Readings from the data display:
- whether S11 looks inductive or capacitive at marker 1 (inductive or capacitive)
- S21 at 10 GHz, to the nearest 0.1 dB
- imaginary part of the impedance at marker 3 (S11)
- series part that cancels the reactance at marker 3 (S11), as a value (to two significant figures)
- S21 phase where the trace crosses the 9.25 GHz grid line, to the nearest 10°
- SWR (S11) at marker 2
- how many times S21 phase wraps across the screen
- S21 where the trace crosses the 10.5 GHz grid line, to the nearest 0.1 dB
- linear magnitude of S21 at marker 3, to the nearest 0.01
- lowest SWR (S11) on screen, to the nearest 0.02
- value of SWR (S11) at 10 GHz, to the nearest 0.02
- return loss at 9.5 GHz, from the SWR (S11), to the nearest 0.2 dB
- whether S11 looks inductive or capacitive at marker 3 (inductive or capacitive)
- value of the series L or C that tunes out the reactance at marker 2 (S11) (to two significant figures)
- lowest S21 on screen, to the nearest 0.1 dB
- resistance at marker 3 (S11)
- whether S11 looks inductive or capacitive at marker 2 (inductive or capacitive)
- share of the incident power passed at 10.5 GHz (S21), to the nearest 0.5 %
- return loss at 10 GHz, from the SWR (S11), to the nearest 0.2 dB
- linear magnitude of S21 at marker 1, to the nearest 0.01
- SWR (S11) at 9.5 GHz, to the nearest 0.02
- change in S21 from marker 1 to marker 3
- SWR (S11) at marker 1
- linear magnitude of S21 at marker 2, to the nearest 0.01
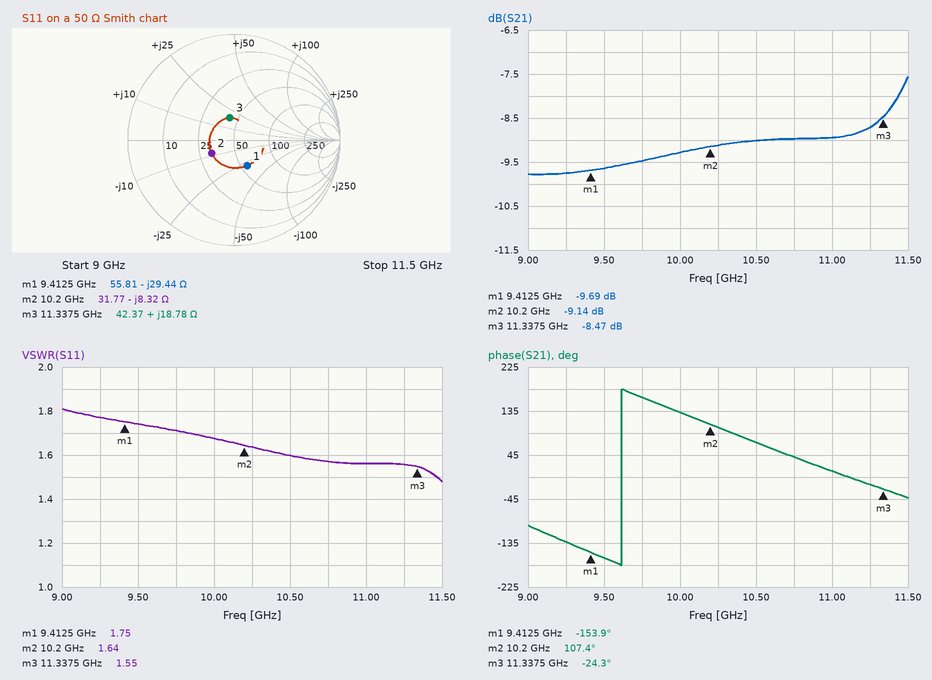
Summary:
capacitive
-9.3 dB
+18.78 Ω
750 fF
-130°
1.64
1
-9.0 dB
0.38
1.48
1.68
11.4 dB
inductive
130 pH
-9.8 dB
42.37 Ω
capacitive
12.5 %
12.0 dB
0.33
1.74
1.22 dB
1.75
0.35
